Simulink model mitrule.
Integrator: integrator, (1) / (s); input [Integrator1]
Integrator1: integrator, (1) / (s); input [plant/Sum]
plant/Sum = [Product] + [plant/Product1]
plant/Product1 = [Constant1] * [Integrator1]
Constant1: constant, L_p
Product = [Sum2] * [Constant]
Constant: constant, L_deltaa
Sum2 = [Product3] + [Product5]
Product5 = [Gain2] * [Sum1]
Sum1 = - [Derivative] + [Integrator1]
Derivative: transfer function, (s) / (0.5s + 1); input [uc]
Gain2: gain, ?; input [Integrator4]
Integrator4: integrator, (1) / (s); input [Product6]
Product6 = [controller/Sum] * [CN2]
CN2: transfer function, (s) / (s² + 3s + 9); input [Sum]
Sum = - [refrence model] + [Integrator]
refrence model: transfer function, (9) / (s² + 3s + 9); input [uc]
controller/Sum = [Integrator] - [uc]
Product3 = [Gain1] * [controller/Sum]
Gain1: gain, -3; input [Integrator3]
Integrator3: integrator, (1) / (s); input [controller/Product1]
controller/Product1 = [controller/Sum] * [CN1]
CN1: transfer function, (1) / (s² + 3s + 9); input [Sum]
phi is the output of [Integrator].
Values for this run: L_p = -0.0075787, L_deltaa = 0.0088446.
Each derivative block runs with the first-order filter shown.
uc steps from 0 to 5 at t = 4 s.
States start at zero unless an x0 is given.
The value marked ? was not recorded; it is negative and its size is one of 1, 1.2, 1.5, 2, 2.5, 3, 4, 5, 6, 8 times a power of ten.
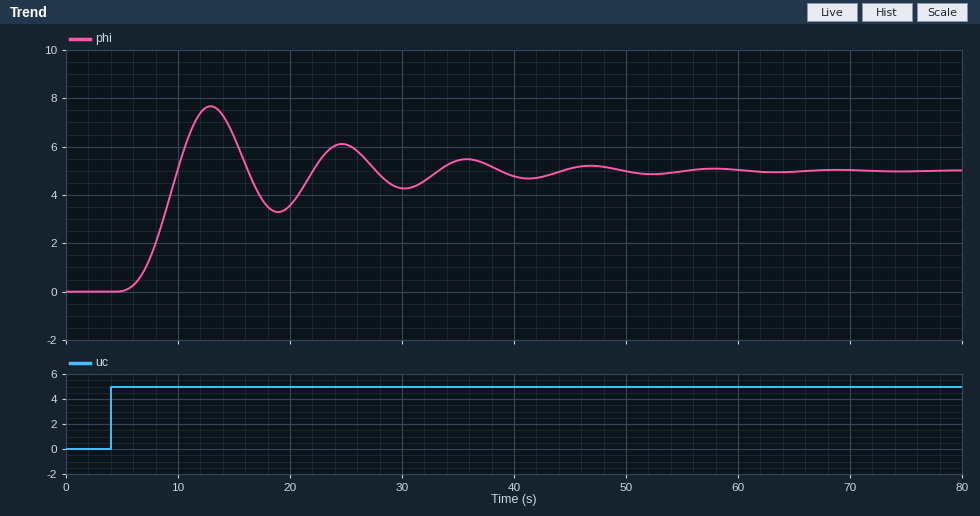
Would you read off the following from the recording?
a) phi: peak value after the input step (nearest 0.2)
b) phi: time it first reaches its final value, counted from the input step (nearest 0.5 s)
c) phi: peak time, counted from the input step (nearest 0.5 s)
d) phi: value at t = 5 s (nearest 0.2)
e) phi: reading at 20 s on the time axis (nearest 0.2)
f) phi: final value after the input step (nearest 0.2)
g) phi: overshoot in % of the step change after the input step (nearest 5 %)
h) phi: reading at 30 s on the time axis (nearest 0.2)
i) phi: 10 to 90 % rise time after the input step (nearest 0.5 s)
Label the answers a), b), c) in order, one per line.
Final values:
a) 7.6
b) 6.0 s
c) 9.0 s
d) 0.0
e) 3.6
f) 5.0
g) 55 %
h) 4.2
i) 3.0 s
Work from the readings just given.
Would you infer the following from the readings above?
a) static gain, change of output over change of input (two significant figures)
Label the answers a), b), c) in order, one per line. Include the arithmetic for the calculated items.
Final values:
a) (5 - 0) / (5 - 0) = 1.0
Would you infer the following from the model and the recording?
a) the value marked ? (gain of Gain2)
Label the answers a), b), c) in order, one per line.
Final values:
a) -8
